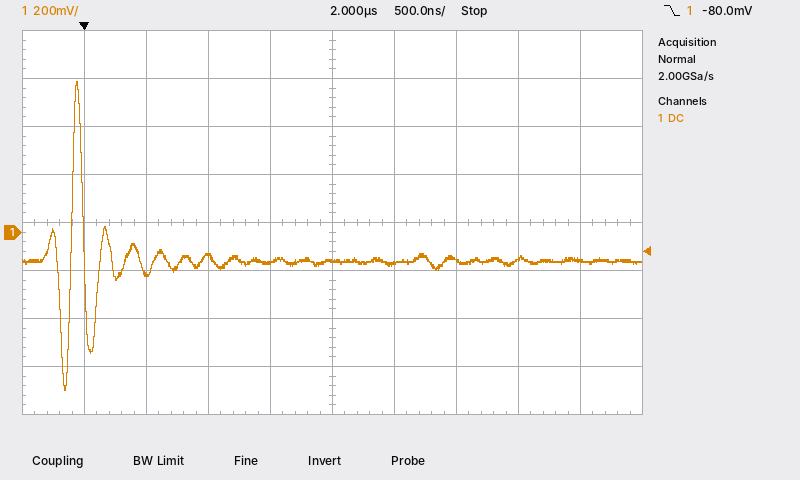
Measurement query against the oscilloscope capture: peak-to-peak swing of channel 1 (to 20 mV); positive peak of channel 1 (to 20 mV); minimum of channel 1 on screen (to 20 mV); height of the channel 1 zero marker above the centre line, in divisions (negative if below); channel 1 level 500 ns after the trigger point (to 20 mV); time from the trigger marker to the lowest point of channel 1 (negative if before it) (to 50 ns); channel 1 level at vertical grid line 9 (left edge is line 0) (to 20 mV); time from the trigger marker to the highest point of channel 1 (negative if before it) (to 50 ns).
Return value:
1.28 V
620 mV
-660 mV
-0.2 div
-180 mV
-150 ns
-120 mV
-50 ns
